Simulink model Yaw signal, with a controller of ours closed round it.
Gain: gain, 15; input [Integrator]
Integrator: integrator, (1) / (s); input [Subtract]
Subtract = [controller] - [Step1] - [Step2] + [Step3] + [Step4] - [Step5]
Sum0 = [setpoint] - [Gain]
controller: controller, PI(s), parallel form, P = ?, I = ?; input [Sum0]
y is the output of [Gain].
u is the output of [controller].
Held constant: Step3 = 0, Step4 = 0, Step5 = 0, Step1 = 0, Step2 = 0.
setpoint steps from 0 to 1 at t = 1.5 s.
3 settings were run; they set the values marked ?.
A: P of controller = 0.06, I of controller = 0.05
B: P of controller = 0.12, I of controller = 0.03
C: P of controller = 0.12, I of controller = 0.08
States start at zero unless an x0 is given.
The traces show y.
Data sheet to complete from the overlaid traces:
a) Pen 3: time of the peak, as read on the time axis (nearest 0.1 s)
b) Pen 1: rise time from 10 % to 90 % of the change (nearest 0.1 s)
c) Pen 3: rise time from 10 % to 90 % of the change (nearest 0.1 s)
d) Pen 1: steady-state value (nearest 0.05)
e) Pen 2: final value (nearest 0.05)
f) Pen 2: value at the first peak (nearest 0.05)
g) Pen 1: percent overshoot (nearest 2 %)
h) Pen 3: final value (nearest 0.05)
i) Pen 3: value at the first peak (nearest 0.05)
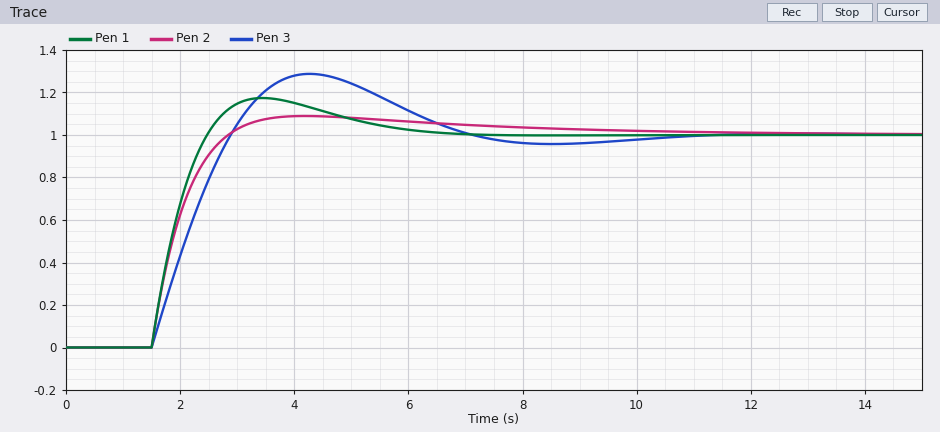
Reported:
4.3 s
0.7 s
1.1 s
1.00
1.00
1.10
18 %
1.00
1.30
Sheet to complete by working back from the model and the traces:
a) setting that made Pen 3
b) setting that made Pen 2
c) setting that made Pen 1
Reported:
A
B
C
